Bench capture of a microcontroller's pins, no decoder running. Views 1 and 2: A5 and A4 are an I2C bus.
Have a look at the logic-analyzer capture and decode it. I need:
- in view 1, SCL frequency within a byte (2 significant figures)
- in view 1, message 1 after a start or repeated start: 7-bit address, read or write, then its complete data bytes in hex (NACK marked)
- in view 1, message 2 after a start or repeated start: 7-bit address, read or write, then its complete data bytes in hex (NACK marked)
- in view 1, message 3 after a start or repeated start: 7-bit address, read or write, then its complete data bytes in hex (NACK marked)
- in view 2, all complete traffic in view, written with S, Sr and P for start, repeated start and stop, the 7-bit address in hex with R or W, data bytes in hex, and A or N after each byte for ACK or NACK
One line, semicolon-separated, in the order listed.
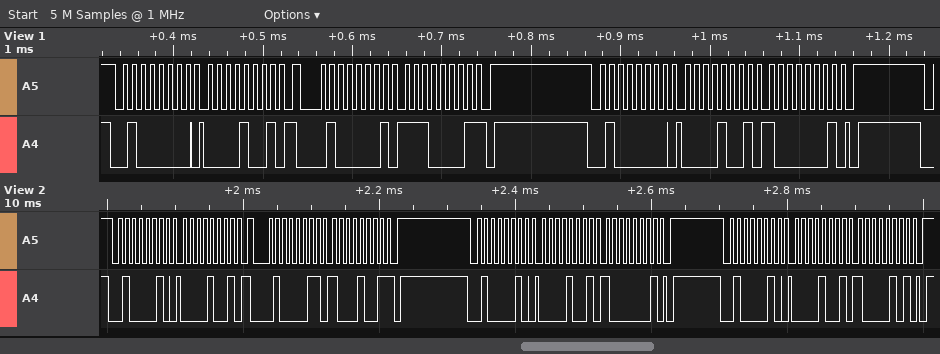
100 kHz; 0x20 write: 09; 0x20 read: E1 NACK; 0x20 write: 09 81; S 21W A 09 A Sr 21R A 89 N P S 21W A 09 A 81 A P S 21W A 09 A 85 A P
